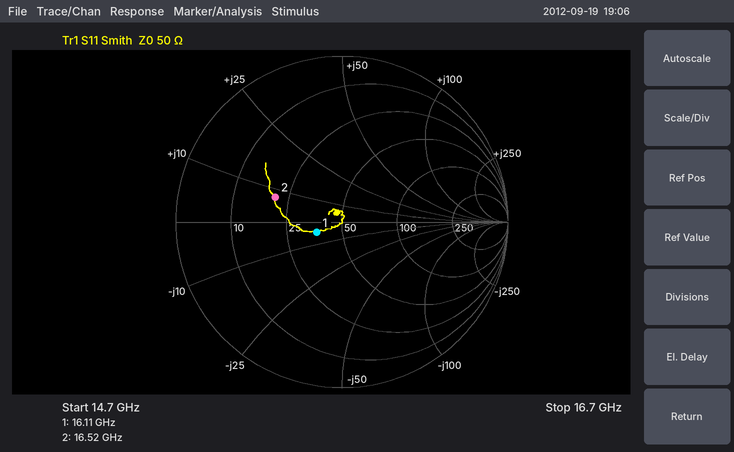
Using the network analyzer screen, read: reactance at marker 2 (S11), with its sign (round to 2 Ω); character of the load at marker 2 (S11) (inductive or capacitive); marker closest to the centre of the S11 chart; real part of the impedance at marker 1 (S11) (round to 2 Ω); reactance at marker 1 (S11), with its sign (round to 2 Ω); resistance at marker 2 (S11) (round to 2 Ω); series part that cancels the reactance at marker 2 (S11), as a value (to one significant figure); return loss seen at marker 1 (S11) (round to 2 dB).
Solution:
+8 Ω
inductive
marker 1
36 Ω
-4 Ω
20 Ω
1 pF
16 dB
